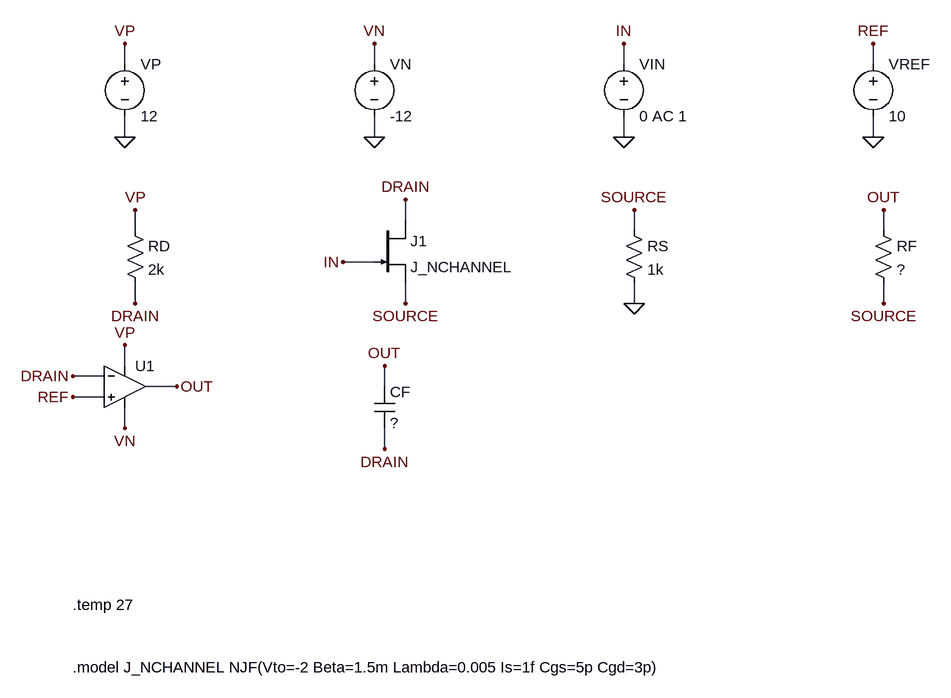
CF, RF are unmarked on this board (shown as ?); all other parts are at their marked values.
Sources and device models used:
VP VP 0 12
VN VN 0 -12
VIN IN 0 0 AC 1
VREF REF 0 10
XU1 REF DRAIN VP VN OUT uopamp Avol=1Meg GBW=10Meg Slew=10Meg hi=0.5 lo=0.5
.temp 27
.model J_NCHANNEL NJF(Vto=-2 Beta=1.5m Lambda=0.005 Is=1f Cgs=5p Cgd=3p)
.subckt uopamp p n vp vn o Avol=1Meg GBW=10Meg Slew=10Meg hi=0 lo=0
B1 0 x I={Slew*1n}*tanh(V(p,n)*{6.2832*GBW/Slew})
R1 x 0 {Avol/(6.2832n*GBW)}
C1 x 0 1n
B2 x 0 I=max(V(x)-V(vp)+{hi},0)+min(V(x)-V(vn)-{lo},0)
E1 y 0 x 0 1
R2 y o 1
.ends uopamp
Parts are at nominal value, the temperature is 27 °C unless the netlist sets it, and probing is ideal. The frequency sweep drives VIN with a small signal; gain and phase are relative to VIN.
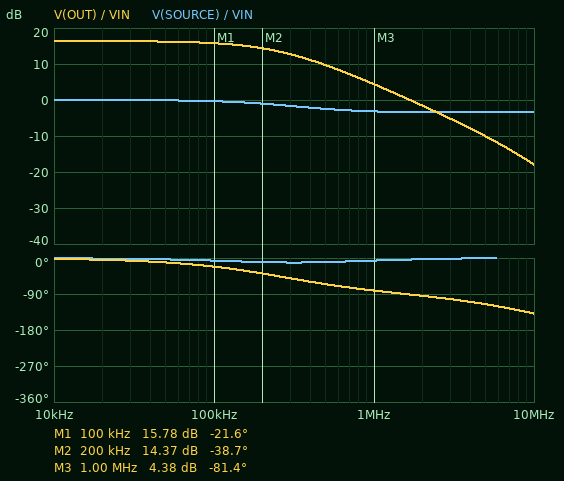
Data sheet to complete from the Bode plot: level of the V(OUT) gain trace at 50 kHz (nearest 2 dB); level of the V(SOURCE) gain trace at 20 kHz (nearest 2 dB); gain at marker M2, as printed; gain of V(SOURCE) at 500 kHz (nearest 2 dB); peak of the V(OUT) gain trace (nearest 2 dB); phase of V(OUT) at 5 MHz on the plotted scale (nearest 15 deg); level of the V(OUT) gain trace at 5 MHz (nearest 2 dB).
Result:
16 dB
0 dB
14.37 dB
-2 dB
16 dB
-120 deg
-10 dB
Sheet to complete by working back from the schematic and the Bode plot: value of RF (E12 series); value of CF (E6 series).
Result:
5.6 kΩ
68 pF
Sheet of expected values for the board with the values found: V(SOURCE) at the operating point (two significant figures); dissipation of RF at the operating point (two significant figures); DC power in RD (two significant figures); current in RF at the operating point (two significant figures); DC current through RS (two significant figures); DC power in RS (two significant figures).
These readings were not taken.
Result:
1.2 V
230 µW
2.0 mW
200 µA
1.2 mA
1.4 mW
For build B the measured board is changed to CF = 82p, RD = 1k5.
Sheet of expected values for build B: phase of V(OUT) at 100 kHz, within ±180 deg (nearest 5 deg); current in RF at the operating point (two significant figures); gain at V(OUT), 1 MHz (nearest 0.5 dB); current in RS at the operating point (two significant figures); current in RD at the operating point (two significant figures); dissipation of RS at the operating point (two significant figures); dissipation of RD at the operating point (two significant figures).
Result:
-25 deg
260 µA
3.0 dB
1.1 mA
1.3 mA
1.2 mW
2.7 mW
